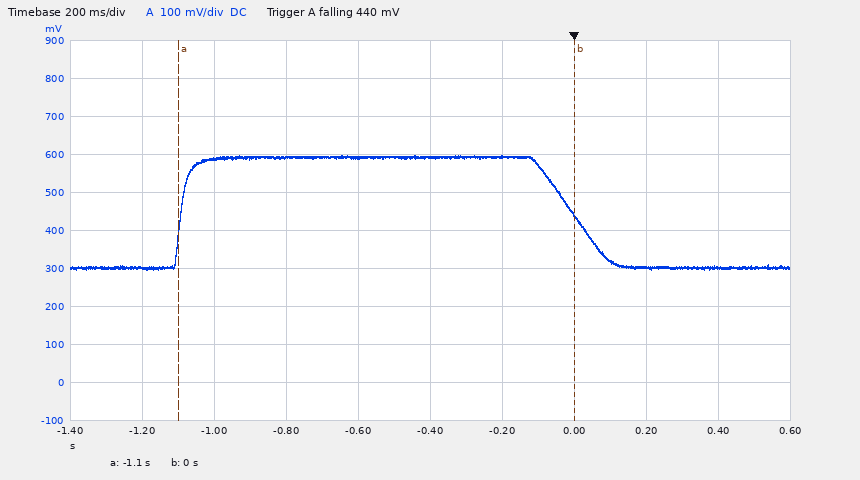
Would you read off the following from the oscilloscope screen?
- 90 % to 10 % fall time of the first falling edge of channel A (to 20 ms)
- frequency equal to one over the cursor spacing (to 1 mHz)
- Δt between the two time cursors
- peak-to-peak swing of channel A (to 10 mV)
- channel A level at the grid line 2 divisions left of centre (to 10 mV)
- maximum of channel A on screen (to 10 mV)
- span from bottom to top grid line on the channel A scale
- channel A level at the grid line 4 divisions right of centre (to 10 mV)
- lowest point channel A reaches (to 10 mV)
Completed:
180 ms
909 mHz
1.10 s
300 mV
590 mV
600 mV
1 V
300 mV
300 mV
